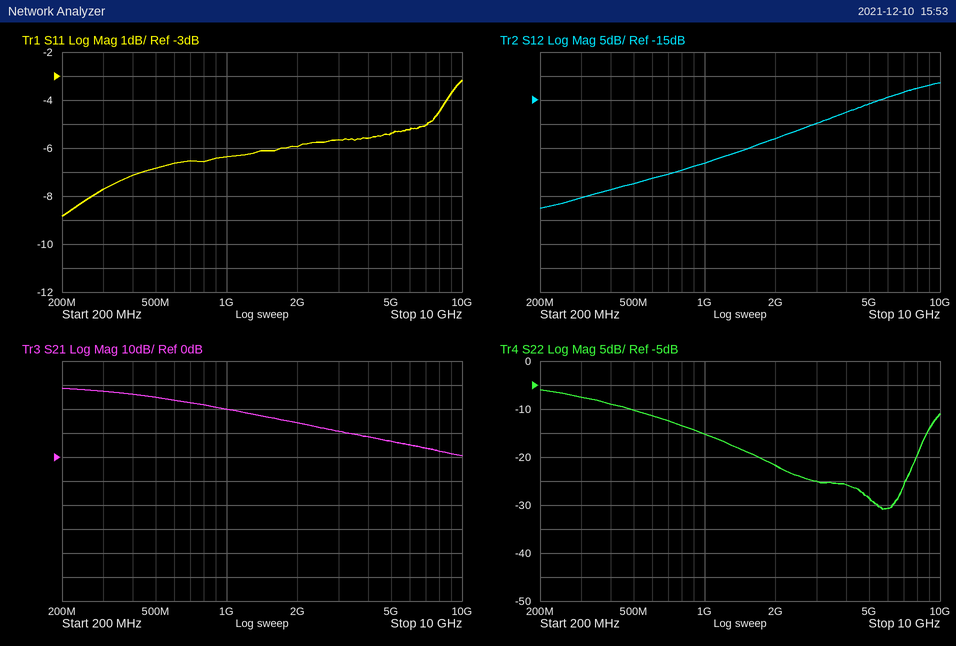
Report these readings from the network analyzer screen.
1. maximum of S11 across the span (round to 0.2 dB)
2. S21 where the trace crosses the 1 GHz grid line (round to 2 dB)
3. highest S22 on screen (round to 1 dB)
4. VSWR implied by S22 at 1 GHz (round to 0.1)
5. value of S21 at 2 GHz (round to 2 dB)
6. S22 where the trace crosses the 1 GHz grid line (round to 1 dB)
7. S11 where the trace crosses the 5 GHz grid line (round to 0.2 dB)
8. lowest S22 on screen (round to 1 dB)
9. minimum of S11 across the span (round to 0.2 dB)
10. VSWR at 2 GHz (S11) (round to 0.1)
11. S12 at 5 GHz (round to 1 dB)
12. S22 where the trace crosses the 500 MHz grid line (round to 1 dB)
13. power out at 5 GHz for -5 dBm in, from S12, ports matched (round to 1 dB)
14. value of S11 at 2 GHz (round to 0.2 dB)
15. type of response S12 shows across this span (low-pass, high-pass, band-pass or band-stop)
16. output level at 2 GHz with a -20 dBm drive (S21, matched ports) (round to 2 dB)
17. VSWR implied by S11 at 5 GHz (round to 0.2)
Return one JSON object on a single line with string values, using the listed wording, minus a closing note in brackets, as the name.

{"maximum of S11 across the span": "-3.2 dB", "S21 where the trace crosses the 1 GHz grid line": "20 dB", "highest S22 on screen": "-6 dB", "VSWR implied by S22 at 1 GHz": "1.4", "value of S21 at 2 GHz": "14 dB", "S22 where the trace crosses the 1 GHz grid line": "-15 dB", "S11 where the trace crosses the 5 GHz grid line": "-5.4 dB", "lowest S22 on screen": "-31 dB", "minimum of S11 across the span": "-8.8 dB", "VSWR at 2 GHz (S11)": "3.0", "S12 at 5 GHz": "-16 dB", "S22 where the trace crosses the 500 MHz grid line": "-10 dB", "power out at 5 GHz for -5 dBm in, from S12, ports matched": "-21 dBm", "value of S11 at 2 GHz": "-6.0 dB", "type of response S12 shows across this span": "high-pass", "output level at 2 GHz with a -20 dBm drive (S21, matched ports)": "-6 dBm", "VSWR implied by S11 at 5 GHz": "3.4"}
